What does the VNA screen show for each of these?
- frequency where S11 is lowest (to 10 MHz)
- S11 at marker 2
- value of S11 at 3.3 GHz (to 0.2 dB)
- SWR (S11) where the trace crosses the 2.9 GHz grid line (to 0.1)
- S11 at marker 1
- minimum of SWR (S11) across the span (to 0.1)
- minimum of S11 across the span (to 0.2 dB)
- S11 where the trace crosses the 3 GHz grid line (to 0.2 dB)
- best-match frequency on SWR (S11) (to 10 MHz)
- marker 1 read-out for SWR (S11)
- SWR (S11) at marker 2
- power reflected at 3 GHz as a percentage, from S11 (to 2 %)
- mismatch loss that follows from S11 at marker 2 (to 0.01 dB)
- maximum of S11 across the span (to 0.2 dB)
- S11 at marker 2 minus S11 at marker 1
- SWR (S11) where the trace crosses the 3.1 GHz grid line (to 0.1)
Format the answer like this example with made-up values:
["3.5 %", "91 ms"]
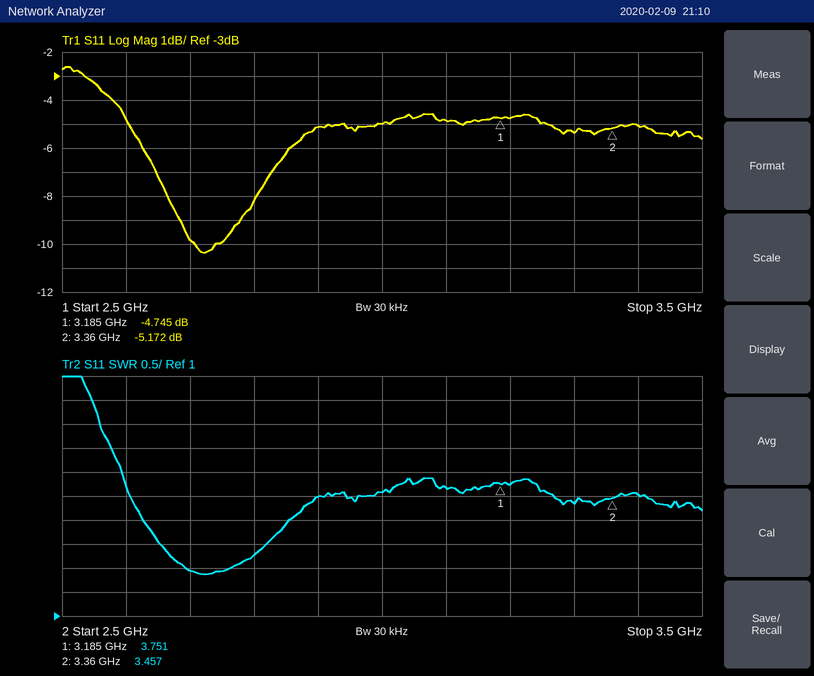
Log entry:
["2.72 GHz", "-5.172 dB", "-5.4 dB", "3.5", "-4.745 dB", "1.9", "-10.4 dB", "-5.0 dB", "2.72 GHz", "3.751", "3.457", "32 %", "1.57 dB", "-2.6 dB", "-0.427 dB", "3.7"]
